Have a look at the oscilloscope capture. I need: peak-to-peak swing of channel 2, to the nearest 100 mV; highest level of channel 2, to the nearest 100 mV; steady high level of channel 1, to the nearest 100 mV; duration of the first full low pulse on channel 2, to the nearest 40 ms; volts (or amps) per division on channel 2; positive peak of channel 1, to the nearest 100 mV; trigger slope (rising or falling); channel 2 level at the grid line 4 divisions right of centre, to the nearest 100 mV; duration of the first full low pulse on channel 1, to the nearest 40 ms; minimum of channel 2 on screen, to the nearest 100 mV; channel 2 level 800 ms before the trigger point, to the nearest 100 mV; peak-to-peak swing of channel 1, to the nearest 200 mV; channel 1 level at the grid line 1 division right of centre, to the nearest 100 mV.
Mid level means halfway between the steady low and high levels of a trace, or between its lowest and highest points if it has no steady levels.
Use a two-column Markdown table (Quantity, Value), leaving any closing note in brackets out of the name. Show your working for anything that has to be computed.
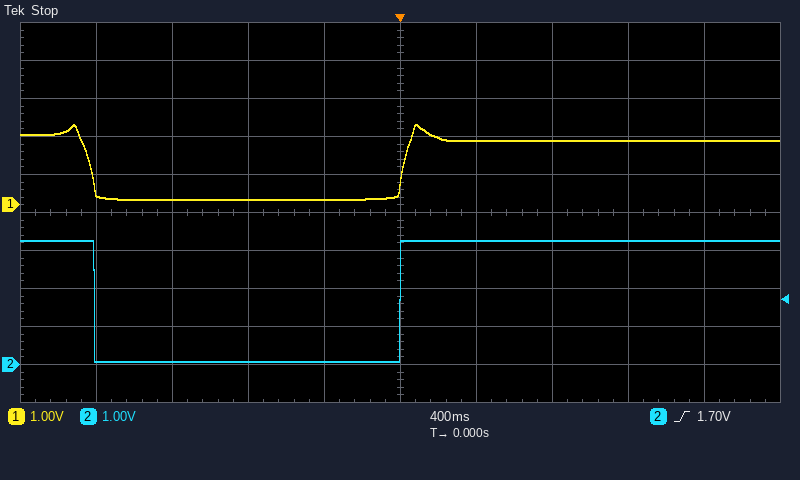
| Quantity | Value |
|---|---|
| peak-to-peak swing of channel 2, to the nearest 100 mV | 3.3 V − (100 mV) = 3.2 V |
| highest level of channel 2, to the nearest 100 mV | 3.3 V |
| steady high level of channel 1, to the nearest 100 mV | 1.7 V |
| duration of the first full low pulse on channel 2, to the nearest 40 ms | 1.60 s |
| volts (or amps) per division on channel 2 | 1 V |
| positive peak of channel 1, to the nearest 100 mV | 2.1 V |
| trigger slope | rising |
| channel 2 level at the grid line 4 divisions right of centre, to the nearest 100 mV | 3.3 V |
| duration of the first full low pulse on channel 1, to the nearest 40 ms | 1.64 s |
| minimum of channel 2 on screen, to the nearest 100 mV | 100 mV |
| channel 2 level 800 ms before the trigger point, to the nearest 100 mV | 100 mV |
| peak-to-peak swing of channel 1, to the nearest 200 mV | 2.0 V |
| channel 1 level at the grid line 1 division right of centre, to the nearest 100 mV | 1.7 V |
